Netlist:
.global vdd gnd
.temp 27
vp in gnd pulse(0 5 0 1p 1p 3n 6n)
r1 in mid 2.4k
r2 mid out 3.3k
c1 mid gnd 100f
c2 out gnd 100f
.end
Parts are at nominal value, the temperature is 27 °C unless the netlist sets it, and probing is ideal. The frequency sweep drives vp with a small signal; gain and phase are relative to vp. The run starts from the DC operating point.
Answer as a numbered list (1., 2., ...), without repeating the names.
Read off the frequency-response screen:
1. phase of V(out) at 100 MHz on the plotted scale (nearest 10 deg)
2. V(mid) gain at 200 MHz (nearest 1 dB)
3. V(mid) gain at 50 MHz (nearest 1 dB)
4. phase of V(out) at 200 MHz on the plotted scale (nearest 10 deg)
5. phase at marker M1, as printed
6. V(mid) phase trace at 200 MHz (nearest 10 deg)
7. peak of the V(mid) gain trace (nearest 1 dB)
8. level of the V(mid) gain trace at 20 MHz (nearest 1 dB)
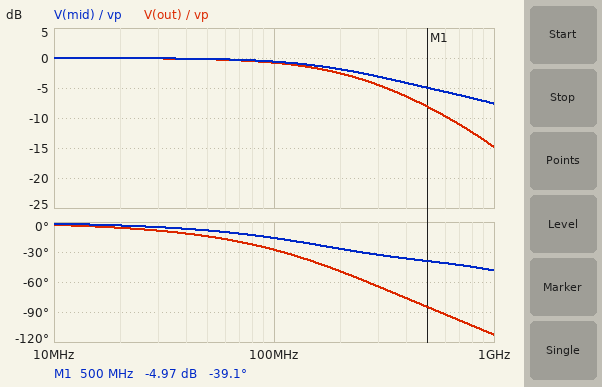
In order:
1. -30 deg
2. -2 dB
3. 0 dB
4. -50 deg
5. -39.1 deg
6. -30 deg
7. 0 dB
8. 0 dB
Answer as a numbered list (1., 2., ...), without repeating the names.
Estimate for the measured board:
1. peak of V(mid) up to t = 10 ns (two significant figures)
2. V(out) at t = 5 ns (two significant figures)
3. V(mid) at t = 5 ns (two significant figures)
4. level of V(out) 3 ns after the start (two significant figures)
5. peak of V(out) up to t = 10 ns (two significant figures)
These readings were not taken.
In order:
1. 5.0 V
2. 330 mV
3. 180 mV
4. 4.9 V
5. 4.9 V
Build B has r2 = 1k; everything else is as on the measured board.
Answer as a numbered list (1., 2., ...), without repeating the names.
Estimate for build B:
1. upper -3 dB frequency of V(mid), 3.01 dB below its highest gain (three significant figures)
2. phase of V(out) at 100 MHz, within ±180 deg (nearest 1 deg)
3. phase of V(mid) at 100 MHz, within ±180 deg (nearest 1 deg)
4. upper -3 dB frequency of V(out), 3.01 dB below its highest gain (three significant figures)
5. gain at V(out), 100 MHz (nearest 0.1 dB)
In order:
1. 306 MHz
2. -20 deg
3. -17 deg
4. 295 MHz
5. -0.5 dB
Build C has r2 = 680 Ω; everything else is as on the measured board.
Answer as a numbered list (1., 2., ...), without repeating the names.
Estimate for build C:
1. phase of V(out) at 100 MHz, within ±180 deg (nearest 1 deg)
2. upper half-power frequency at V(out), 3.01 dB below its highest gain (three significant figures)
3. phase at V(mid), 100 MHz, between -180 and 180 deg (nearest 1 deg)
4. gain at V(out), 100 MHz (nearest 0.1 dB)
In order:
1. -19 deg
2. 307 MHz
3. -17 deg
4. -0.4 dB
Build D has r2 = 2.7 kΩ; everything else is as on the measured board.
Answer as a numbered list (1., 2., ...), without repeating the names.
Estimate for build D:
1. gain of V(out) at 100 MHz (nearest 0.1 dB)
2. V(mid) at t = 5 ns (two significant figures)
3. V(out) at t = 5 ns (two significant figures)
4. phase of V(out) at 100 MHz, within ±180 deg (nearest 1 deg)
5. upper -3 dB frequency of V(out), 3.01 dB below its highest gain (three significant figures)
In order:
1. -0.7 dB
2. 160 mV
3. 270 mV
4. -26 deg
5. 239 MHz
